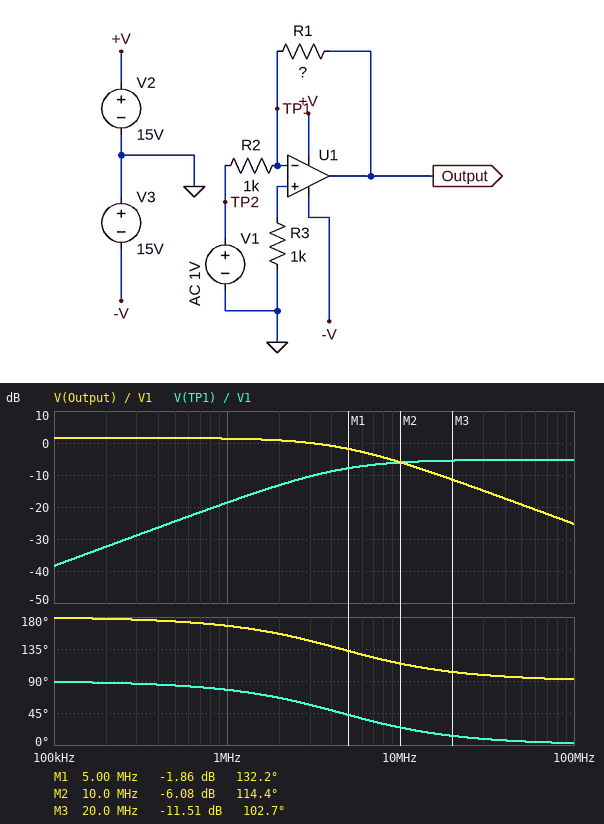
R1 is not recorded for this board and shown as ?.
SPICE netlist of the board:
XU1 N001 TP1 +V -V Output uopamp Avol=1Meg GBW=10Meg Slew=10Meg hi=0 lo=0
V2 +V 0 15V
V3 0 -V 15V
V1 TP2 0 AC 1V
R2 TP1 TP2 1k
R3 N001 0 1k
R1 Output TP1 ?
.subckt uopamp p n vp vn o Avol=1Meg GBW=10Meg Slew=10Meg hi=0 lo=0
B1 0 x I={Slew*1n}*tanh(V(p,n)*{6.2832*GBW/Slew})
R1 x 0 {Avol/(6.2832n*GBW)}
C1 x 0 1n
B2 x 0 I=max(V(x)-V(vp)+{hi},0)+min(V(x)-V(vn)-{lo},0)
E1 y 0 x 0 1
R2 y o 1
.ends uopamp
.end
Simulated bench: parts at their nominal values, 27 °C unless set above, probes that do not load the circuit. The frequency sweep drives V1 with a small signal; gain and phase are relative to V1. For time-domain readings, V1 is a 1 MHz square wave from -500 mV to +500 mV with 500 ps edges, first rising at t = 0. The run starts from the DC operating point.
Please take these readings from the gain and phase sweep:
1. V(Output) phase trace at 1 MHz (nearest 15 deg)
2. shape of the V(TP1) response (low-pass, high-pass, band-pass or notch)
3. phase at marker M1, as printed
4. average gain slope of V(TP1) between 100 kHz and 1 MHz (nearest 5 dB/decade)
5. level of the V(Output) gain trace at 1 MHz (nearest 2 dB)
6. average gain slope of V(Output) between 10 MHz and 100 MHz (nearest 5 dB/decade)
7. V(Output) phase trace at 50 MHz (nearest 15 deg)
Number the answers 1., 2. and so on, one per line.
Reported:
1. 165 deg
2. high-pass
3. 132.2 deg
4. 20 dB/decade
5. 2 dB
6. -20 dB/decade
7. 90 deg
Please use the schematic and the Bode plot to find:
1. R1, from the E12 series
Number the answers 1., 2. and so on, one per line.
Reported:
1. 1.2 kΩ
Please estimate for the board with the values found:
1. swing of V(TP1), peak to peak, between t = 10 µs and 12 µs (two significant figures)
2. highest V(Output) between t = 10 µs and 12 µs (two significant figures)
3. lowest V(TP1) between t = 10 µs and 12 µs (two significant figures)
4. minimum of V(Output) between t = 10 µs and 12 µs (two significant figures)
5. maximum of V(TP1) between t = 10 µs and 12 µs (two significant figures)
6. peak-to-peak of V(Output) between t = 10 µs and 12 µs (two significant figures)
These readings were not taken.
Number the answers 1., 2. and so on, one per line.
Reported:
1. 1.1 V
2. 600 mV
3. -540 mV
4. -600 mV
5. 540 mV
6. 1.2 V
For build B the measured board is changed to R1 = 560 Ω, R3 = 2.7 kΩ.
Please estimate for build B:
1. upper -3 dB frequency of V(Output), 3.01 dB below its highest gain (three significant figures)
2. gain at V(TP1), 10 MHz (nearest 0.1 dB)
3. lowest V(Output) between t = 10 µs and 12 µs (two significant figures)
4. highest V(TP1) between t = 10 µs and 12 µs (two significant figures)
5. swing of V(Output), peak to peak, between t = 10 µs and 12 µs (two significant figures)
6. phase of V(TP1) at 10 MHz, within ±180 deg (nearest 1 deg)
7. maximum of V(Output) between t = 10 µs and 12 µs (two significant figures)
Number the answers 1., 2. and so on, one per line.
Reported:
1. 6.41 MHz
2. -10.4 dB
3. -280 mV
4. 360 mV
5. 560 mV
6. 33 deg
7. 280 mV
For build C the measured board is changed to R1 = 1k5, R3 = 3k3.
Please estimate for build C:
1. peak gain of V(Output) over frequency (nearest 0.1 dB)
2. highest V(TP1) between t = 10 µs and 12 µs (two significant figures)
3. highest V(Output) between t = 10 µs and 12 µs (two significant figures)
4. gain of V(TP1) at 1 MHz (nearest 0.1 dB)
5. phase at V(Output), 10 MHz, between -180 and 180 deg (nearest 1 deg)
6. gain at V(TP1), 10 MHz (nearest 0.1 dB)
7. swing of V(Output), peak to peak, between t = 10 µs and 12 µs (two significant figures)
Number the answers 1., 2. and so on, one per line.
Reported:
1. 3.5 dB
2. 600 mV
3. 750 mV
4. -16.7 dB
5. 112 deg
6. -5.1 dB
7. 1.5 V
